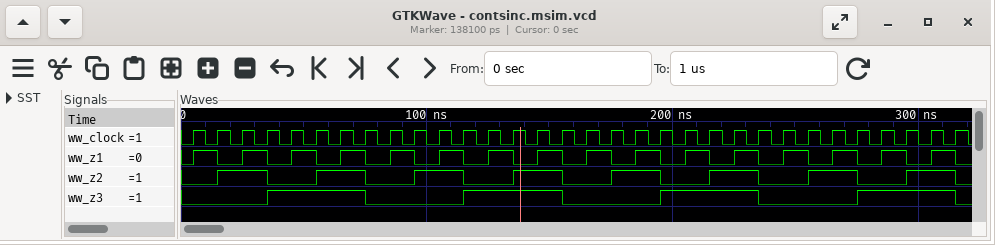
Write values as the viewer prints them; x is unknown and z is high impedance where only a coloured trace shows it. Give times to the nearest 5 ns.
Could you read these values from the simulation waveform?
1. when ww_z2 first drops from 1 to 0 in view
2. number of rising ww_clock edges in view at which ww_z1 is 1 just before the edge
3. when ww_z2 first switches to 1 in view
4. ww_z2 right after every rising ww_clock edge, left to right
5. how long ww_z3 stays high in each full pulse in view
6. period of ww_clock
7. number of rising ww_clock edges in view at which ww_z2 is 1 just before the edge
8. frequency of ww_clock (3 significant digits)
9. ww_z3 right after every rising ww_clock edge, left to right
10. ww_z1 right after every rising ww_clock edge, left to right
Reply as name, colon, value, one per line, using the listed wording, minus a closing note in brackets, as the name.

when ww_z2 first drops from 1 to 0 in view: 35 ns
number of rising ww_clock edges in view at which ww_z1 is 1 just before the edge: 16
when ww_z2 first switches to 1 in view: 15 ns
ww_z2 right after every rising ww_clock edge, left to right: 0 1 1 0 0 1 1 0 0 1 1 0 0 1 1 0 0 1 1 0 0 1 1 0 0 1 1 0 0 1 1 0
how long ww_z3 stays high in each full pulse in view: 40 ns, 40 ns, 40 ns, 40 ns
period of ww_clock: 10 ns
number of rising ww_clock edges in view at which ww_z2 is 1 just before the edge: 16
frequency of ww_clock: 100 MHz
ww_z3 right after every rising ww_clock edge, left to right: 0 0 0 1 1 1 1 0 0 0 0 1 1 1 1 0 0 0 0 1 1 1 1 0 0 0 0 1 1 1 1 0
ww_z1 right after every rising ww_clock edge, left to right: 1 0 1 0 1 0 1 0 1 0 1 0 1 0 1 0 1 0 1 0 1 0 1 0 1 0 1 0 1 0 1 0
